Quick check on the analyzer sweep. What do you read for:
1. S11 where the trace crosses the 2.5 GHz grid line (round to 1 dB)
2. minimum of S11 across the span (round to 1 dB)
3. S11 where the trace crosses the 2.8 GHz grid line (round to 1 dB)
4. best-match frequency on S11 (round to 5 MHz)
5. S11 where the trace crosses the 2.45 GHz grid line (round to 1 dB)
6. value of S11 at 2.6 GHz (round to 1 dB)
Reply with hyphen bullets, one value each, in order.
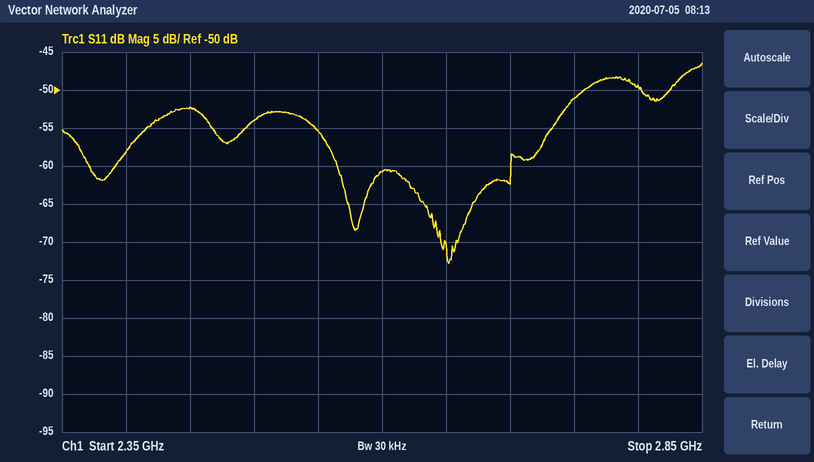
- -54 dB
- -73 dB
- -49 dB
- 2.650 GHz
- -52 dB
- -61 dB
